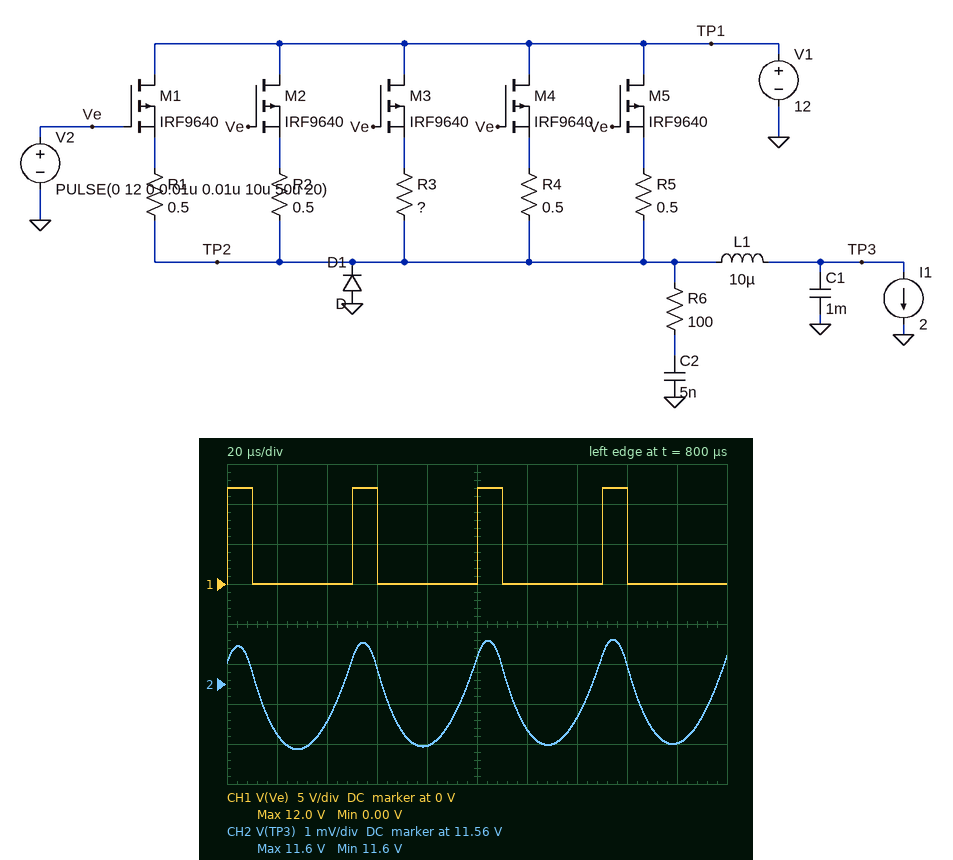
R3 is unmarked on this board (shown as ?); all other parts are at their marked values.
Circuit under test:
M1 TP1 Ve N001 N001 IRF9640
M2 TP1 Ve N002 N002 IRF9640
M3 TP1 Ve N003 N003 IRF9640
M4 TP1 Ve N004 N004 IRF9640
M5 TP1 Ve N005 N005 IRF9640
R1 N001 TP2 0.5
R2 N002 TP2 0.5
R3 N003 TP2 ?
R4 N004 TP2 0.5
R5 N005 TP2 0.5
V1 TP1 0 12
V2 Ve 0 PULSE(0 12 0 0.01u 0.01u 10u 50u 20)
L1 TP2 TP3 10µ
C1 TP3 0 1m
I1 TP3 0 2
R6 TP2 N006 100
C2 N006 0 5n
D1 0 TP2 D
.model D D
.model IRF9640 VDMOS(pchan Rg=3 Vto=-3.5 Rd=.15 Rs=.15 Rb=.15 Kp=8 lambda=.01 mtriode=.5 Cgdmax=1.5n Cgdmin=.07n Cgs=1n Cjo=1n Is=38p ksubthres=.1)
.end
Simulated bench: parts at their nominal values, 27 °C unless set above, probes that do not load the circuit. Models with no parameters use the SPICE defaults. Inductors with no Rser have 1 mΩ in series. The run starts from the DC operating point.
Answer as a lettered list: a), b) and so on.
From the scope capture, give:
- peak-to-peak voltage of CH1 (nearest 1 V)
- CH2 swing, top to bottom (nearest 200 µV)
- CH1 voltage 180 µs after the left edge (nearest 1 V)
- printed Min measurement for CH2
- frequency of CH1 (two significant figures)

a) 12 V
b) 2.8 mV
c) 0 V
d) 11.6 V
e) 20 kHz
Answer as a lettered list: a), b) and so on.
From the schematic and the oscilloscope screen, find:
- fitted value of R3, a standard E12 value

a) 0.56 Ω
